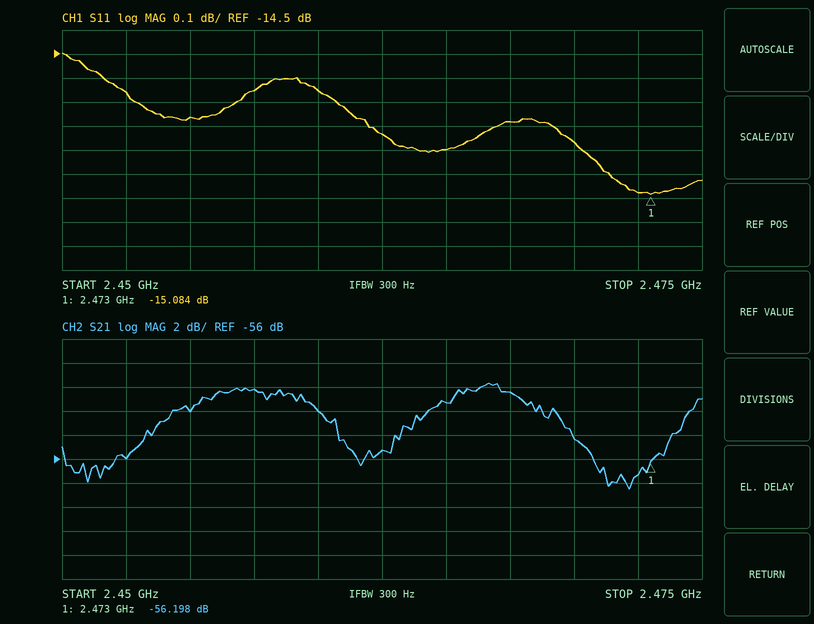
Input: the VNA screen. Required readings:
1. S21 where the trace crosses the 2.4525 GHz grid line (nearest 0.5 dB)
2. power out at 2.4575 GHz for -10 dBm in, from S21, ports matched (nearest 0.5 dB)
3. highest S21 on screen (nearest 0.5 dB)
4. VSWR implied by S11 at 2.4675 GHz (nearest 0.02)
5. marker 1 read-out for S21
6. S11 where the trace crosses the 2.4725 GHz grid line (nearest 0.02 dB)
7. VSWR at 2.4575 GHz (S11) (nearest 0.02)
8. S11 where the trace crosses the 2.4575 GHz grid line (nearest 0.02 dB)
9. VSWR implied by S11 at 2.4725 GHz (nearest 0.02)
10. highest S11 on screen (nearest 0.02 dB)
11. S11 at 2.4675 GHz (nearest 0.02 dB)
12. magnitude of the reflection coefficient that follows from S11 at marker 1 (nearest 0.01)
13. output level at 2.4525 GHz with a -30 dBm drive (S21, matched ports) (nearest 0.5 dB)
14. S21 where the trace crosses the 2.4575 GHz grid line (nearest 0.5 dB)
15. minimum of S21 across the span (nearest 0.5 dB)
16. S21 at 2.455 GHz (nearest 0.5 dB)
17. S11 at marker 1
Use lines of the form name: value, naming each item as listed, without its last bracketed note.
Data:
S21 where the trace crosses the 2.4525 GHz grid line: -56.0 dB
power out at 2.4575 GHz for -10 dBm in, from S21, ports matched: -60.0 dBm
highest S21 on screen: -49.5 dB
VSWR implied by S11 at 2.4675 GHz: 1.44
marker 1 read-out for S21: -56.198 dB
S11 where the trace crosses the 2.4725 GHz grid line: -15.08 dB
VSWR at 2.4575 GHz (S11): 1.46
S11 where the trace crosses the 2.4575 GHz grid line: -14.66 dB
VSWR implied by S11 at 2.4725 GHz: 1.42
highest S11 on screen: -14.50 dB
S11 at 2.4675 GHz: -14.78 dB
magnitude of the reflection coefficient that follows from S11 at marker 1: 0.18
output level at 2.4525 GHz with a -30 dBm drive (S21, matched ports): -86.0 dBm
S21 where the trace crosses the 2.4575 GHz grid line: -50.0 dB
minimum of S21 across the span: -58.5 dB
S21 at 2.455 GHz: -52.0 dB
S11 at marker 1: -15.084 dB
